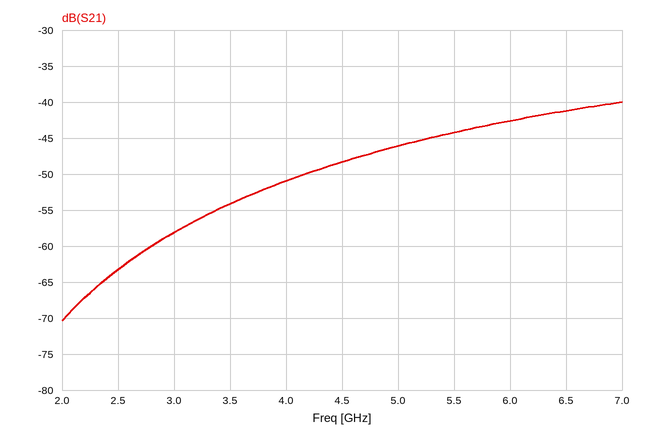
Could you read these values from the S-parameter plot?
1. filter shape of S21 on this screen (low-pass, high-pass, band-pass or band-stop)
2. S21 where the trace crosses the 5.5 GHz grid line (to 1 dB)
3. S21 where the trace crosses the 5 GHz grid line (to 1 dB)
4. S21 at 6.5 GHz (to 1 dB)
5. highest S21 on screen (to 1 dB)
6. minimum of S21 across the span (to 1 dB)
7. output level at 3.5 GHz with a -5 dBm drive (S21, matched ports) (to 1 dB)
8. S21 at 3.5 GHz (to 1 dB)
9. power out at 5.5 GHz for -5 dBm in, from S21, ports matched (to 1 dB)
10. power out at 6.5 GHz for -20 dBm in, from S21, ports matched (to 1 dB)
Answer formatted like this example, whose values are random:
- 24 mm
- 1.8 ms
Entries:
- high-pass
- -44 dB
- -46 dB
- -41 dB
- -40 dB
- -70 dB
- -59 dBm
- -54 dB
- -49 dBm
- -61 dBm
